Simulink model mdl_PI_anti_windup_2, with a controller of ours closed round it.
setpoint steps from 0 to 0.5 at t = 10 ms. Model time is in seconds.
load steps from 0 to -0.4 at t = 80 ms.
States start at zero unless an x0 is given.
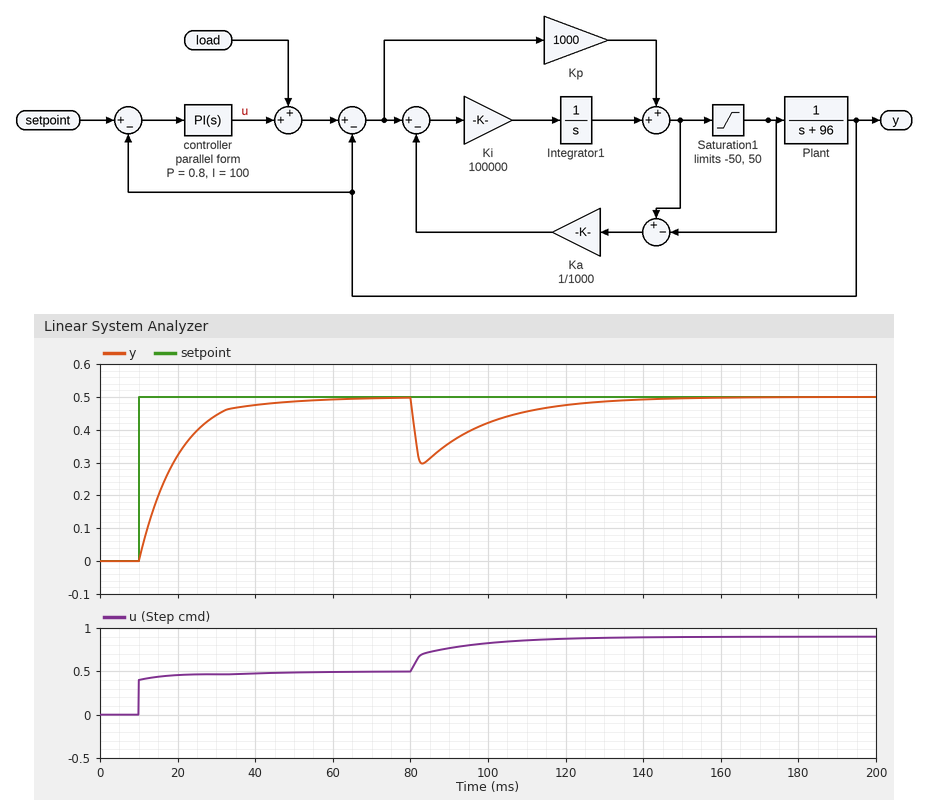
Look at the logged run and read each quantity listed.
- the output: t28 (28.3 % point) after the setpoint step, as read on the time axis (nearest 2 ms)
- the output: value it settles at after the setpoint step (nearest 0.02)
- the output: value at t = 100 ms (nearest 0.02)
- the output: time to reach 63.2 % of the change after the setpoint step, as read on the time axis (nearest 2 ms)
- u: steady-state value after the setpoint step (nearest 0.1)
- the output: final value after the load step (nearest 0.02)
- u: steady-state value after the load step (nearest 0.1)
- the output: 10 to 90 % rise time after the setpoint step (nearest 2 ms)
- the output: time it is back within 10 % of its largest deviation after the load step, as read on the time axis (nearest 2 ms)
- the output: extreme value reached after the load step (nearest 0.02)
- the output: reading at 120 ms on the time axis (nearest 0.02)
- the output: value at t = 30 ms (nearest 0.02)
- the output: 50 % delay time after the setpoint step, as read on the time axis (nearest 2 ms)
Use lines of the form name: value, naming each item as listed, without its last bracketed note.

the output: t28 (28.3 % point) after the setpoint step, as read on the time axis: 14 ms
the output: value it settles at after the setpoint step: 0.50
the output: value at t = 100 ms: 0.42
the output: time to reach 63.2 % of the change after the setpoint step, as read on the time axis: 20 ms
u: steady-state value after the setpoint step: 0.5
the output: final value after the load step: 0.50
u: steady-state value after the load step: 0.9
the output: 10 to 90 % rise time after the setpoint step: 20 ms
the output: time it is back within 10 % of its largest deviation after the load step, as read on the time axis: 124 ms
the output: extreme value reached after the load step: 0.30
the output: reading at 120 ms on the time axis: 0.48
the output: value at t = 30 ms: 0.44
the output: 50 % delay time after the setpoint step, as read on the time axis: 16 ms
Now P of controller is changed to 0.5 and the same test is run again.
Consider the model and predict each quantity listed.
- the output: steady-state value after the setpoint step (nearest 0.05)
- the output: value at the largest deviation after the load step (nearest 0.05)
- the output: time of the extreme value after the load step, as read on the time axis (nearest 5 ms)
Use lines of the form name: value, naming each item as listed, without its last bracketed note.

the output: steady-state value after the setpoint step: 0.50
the output: value at the largest deviation after the load step: 0.25
the output: time of the extreme value after the load step, as read on the time axis: 85 ms
